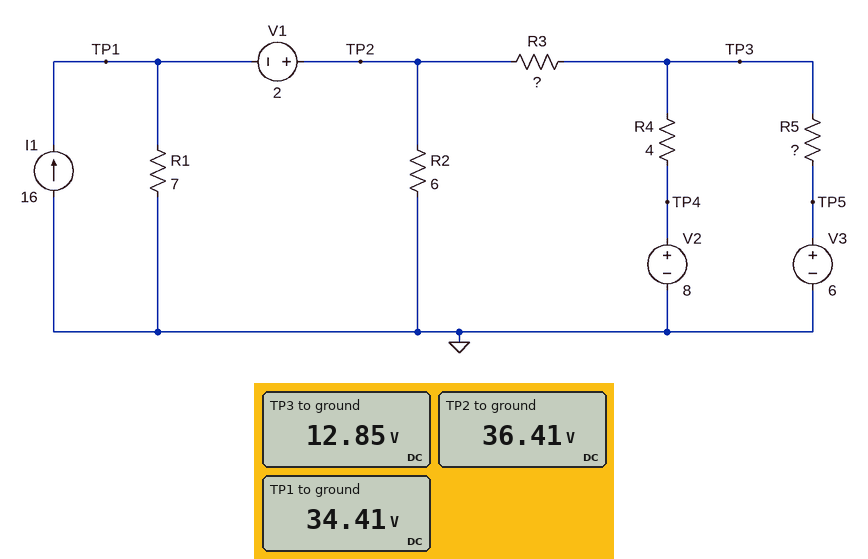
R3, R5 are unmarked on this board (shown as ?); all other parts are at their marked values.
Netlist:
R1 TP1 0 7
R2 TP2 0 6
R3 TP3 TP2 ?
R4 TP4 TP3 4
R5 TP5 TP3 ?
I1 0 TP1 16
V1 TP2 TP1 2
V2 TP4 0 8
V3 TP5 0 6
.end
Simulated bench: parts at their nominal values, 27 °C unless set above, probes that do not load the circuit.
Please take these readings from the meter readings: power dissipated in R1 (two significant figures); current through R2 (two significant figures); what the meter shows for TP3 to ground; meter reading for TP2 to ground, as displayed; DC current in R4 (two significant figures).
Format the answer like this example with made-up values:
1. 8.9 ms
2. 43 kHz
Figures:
1. 170 W
2. 6.1 A
3. 12.85 V
4. 36.41 V
5. 1.2 A
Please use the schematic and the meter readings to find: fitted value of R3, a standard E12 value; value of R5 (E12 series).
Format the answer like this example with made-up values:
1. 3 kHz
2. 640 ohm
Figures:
1. 4.7 Ω
2. 1.8 Ω
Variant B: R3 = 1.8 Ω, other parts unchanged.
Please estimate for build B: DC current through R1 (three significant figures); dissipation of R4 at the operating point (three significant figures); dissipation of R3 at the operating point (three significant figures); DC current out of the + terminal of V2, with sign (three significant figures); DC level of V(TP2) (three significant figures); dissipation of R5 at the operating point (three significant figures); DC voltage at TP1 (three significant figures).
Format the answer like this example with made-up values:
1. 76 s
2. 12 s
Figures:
1. 3.85 A
2. 14.9 W
3. 96.8 W
4. -1.93 A
5. 28.9 V
6. 52.5 W
7. 26.9 V
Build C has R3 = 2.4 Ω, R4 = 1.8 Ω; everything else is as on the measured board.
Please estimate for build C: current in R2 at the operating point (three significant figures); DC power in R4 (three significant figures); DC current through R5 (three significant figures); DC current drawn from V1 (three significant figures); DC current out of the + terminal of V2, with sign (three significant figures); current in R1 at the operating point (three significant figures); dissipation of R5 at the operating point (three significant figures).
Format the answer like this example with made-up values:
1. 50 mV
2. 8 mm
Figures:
1. 5.01 A
2. 15.5 W
3. 4.05 A
4. 12.0 A
5. -2.94 A
6. 4.01 A
7. 29.5 W
